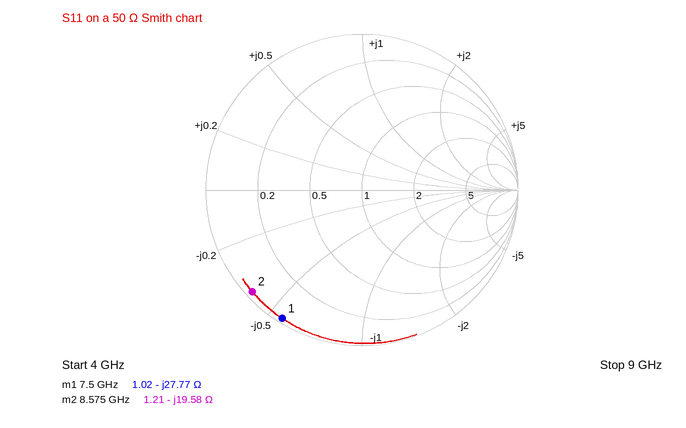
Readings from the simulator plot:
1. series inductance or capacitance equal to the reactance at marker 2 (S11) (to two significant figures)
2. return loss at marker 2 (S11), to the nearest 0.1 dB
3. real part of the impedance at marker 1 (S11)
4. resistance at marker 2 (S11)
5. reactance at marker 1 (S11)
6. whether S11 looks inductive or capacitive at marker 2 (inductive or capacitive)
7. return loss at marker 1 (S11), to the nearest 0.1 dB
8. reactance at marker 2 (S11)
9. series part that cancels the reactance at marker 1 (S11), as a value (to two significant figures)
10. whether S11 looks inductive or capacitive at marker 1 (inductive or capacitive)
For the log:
950 fF
0.4 dB
1.02 Ω
1.21 Ω
-27.77 Ω
capacitive
0.3 dB
-19.58 Ω
590 pH
capacitive
